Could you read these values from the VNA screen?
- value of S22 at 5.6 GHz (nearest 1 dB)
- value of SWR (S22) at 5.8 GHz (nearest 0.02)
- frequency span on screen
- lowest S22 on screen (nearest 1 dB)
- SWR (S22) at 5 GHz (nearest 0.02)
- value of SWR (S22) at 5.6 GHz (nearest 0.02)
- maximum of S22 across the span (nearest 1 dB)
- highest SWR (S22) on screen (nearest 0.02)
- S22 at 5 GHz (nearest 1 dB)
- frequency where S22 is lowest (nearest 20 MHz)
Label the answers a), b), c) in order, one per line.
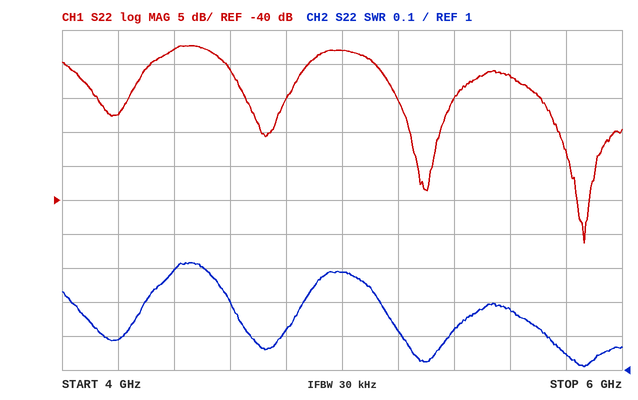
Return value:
a) -22 dB
b) 1.04
c) 2 GHz
d) -46 dB
e) 1.28
f) 1.18
g) -17 dB
h) 1.32
i) -18 dB
j) 5.86 GHz
